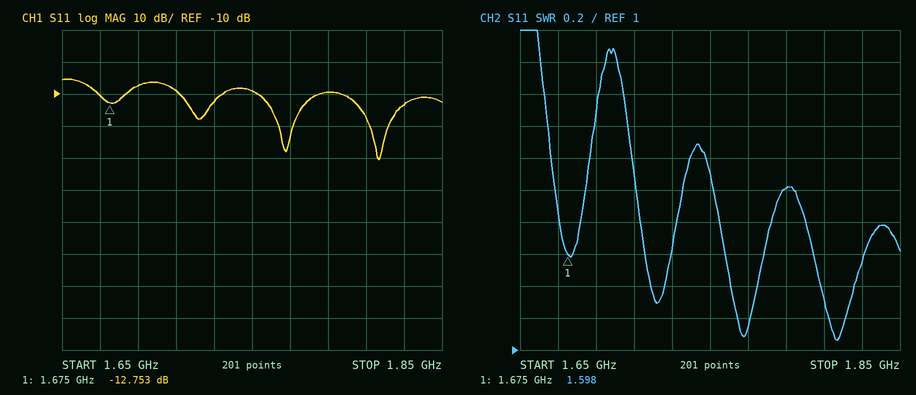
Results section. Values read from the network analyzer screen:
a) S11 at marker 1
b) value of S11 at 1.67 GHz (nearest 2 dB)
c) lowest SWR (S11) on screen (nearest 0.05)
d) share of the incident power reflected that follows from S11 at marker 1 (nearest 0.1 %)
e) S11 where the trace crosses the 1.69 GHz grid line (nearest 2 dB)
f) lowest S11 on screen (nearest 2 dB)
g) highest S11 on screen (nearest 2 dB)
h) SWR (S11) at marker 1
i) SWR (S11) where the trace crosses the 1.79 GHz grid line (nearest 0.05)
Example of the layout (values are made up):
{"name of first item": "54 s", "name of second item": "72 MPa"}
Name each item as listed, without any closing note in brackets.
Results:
{"S11 at marker 1": "-12.753 dB", "value of S11 at 1.67 GHz": "-10 dB", "lowest SWR (S11) on screen": "1.05", "share of the incident power reflected that follows from S11 at marker 1": "5.3 %", "S11 where the trace crosses the 1.69 GHz grid line": "-8 dB", "lowest S11 on screen": "-30 dB", "highest S11 on screen": "-6 dB", "SWR (S11) at marker 1": "1.598", "SWR (S11) where the trace crosses the 1.79 GHz grid line": "2.00"}
